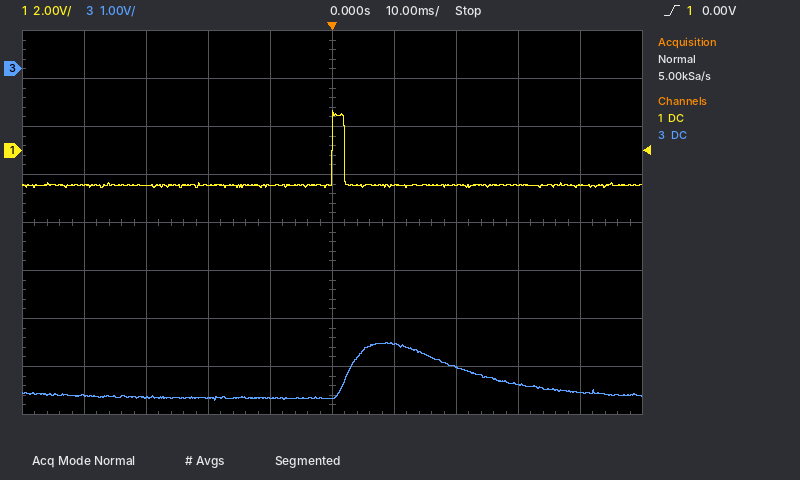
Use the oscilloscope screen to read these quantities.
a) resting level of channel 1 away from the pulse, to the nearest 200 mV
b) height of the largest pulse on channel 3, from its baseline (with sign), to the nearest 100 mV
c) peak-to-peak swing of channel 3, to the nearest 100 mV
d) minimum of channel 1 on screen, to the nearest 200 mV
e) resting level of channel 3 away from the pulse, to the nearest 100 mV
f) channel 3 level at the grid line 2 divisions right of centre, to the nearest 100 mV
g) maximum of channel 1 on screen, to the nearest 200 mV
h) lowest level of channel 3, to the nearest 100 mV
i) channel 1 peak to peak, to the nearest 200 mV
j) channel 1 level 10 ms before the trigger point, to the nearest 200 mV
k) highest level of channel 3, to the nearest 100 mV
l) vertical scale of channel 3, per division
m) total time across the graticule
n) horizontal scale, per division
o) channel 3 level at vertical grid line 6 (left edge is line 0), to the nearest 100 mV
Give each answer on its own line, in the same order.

-1.4 V
+1.1 V
1.2 V
-1.6 V
-6.8 V
-6.2 V
1.6 V
-6.9 V
3.2 V
-1.4 V
-5.7 V
1 V
100 ms
10 ms
-5.7 V
